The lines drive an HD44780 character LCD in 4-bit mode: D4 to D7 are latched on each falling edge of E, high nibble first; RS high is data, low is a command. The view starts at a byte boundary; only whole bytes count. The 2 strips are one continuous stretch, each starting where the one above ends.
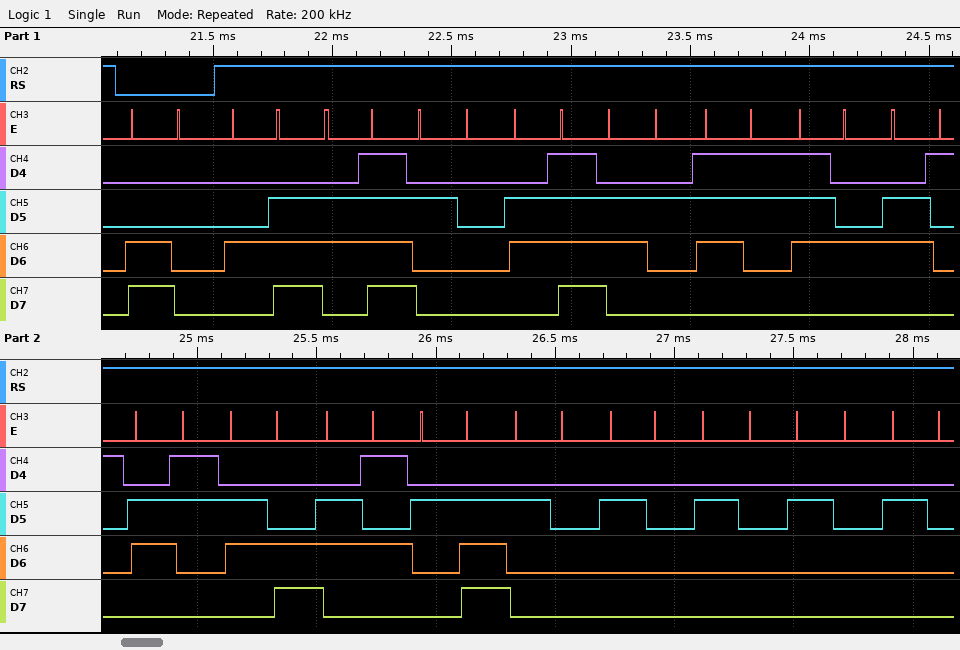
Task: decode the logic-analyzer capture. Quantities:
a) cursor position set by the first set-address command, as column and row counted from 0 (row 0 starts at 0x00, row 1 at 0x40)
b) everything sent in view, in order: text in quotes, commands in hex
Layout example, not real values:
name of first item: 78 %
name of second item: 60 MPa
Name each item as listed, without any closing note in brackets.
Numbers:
cursor position set by the first set-address command, as column and row counted from 0: column 0, row 1
everything sent in view, in order: text in quotes, commands in hex: 0xC0 "No obstacle.     "
